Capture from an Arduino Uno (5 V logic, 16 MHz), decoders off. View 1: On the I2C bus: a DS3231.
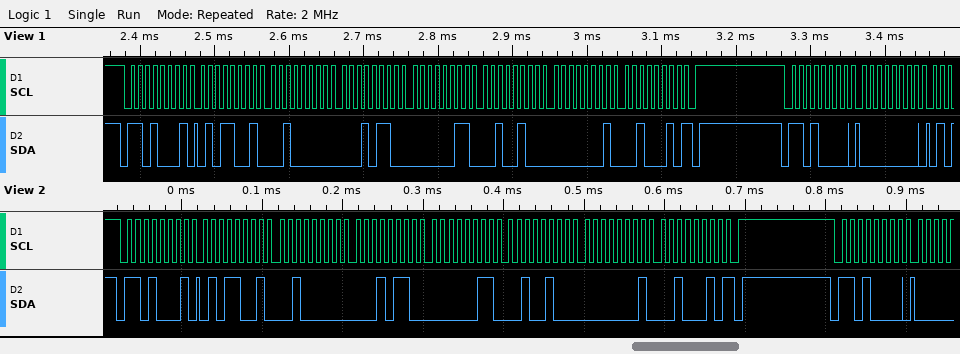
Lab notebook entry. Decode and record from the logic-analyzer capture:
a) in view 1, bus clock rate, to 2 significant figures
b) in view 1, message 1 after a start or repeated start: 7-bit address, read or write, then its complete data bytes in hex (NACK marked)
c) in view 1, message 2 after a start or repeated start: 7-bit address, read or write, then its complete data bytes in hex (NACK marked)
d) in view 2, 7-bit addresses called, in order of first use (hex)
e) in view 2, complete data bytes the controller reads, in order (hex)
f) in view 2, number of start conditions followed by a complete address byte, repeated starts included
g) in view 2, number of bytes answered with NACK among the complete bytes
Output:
100 kHz
0x68 read: 59 20 16 03 24 01 22 NACK
0x68 write: 00
0x68
59 20 16 03 24 01 22
2
1
